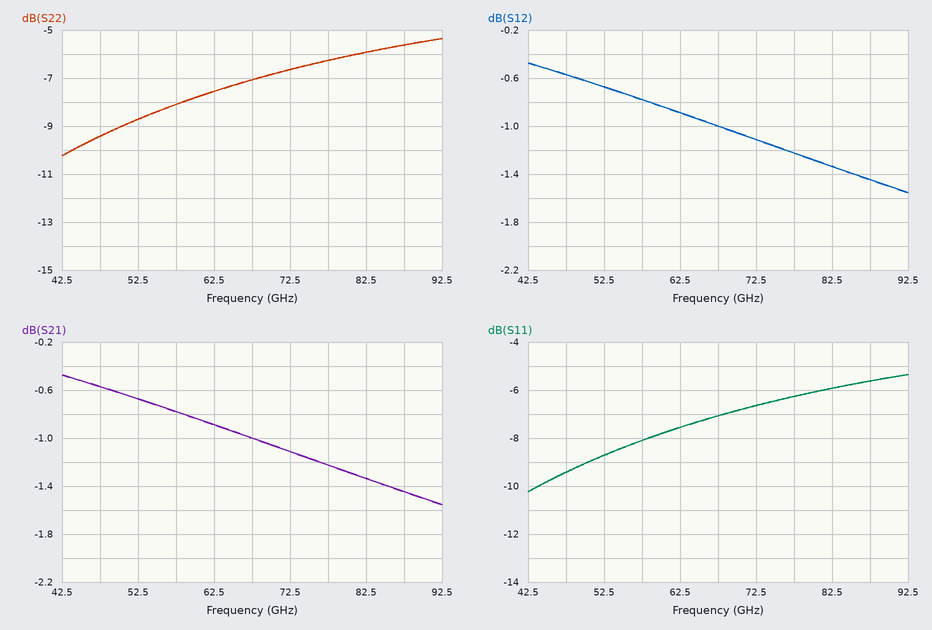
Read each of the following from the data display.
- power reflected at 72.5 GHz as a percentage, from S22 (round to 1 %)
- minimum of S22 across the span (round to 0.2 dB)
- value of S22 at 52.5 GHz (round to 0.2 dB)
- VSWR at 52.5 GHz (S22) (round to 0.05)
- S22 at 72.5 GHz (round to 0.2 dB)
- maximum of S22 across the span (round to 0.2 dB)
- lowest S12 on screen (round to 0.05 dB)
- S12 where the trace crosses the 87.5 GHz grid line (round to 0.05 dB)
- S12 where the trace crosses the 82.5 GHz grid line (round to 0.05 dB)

22 %
-10.2 dB
-8.8 dB
2.15
-6.6 dB
-5.4 dB
-1.55 dB
-1.45 dB
-1.35 dB
